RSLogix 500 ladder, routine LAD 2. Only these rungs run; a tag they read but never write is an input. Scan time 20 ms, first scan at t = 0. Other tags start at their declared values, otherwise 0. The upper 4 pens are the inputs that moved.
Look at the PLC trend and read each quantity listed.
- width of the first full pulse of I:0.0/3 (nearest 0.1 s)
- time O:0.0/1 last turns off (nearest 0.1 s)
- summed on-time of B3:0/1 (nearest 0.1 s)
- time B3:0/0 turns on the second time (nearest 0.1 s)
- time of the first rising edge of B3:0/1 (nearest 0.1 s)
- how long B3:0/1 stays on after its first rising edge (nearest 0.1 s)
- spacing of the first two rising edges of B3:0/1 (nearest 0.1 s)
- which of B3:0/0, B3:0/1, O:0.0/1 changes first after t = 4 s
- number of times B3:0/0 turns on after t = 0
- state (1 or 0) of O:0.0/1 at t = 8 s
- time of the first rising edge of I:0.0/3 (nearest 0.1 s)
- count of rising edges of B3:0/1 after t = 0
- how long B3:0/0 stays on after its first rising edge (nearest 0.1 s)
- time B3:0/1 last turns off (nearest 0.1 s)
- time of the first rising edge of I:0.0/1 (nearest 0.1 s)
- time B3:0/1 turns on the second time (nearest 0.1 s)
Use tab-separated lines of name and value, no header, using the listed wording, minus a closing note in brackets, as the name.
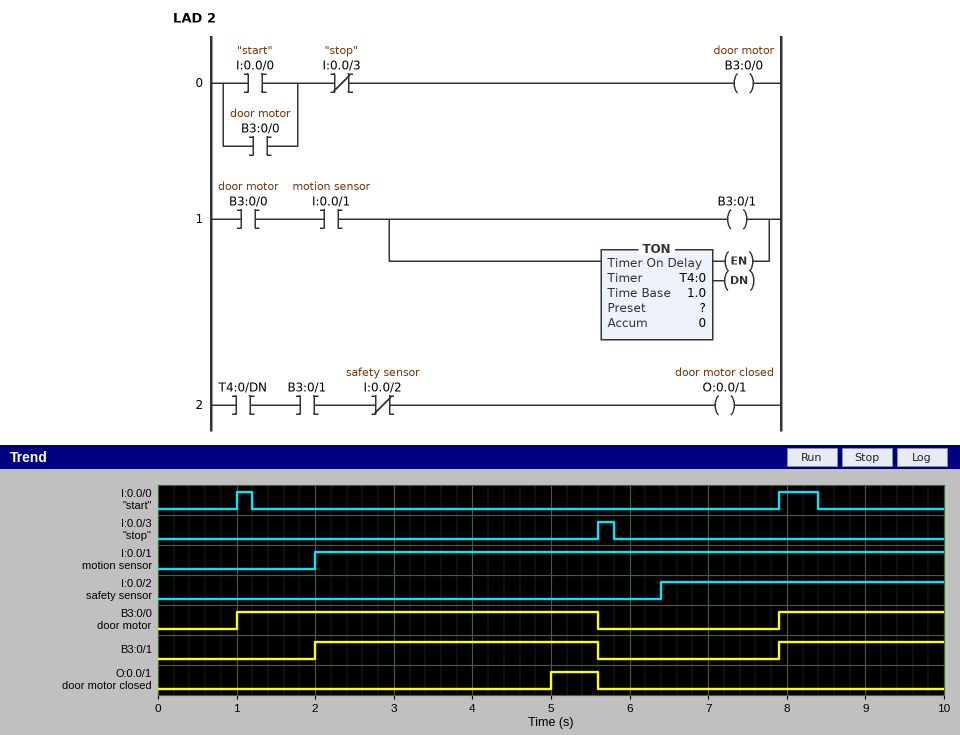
width of the first full pulse of I:0.0/3	0.2 s
time O:0.0/1 last turns off	5.6 s
summed on-time of B3:0/1	5.7 s
time B3:0/0 turns on the second time	7.9 s
time of the first rising edge of B3:0/1	2.0 s
how long B3:0/1 stays on after its first rising edge	3.6 s
spacing of the first two rising edges of B3:0/1	5.9 s
which of B3:0/0, B3:0/1, O:0.0/1 changes first after t = 4 s	O:0.0/1
number of times B3:0/0 turns on after t = 0	2
state (1 or 0) of O:0.0/1 at t = 8 s	0
time of the first rising edge of I:0.0/3	5.6 s
count of rising edges of B3:0/1 after t = 0	2
how long B3:0/0 stays on after its first rising edge	4.6 s
time B3:0/1 last turns off	5.6 s
time of the first rising edge of I:0.0/1	2.0 s
time B3:0/1 turns on the second time	7.9 s
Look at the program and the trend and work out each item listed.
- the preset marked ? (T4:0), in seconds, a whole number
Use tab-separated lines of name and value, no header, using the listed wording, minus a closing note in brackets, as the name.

the preset marked ? (T4:0), in seconds, a whole number	3 s
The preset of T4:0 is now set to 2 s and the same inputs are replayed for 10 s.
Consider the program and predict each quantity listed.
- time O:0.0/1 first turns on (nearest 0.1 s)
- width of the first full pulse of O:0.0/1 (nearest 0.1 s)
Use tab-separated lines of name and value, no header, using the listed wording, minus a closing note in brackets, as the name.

time O:0.0/1 first turns on	4.0 s
width of the first full pulse of O:0.0/1	1.6 s
